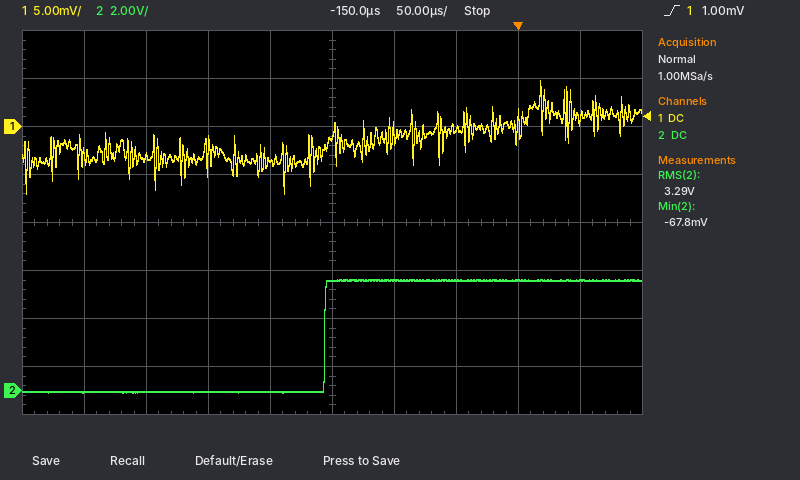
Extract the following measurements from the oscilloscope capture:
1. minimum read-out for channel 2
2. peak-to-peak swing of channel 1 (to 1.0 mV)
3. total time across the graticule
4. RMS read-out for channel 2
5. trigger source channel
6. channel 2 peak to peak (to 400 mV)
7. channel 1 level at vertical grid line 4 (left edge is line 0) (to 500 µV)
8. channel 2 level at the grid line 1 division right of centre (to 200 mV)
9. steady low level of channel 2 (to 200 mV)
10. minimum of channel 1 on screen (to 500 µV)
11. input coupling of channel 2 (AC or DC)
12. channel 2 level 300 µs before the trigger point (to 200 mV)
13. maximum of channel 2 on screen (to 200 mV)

-67.8 mV
12.0 mV
500 µs
3.29 V
channel 1
4.8 V
-3.5 mV
4.6 V
0.0 V
-7.0 mV
DC
0.0 V
4.6 V
